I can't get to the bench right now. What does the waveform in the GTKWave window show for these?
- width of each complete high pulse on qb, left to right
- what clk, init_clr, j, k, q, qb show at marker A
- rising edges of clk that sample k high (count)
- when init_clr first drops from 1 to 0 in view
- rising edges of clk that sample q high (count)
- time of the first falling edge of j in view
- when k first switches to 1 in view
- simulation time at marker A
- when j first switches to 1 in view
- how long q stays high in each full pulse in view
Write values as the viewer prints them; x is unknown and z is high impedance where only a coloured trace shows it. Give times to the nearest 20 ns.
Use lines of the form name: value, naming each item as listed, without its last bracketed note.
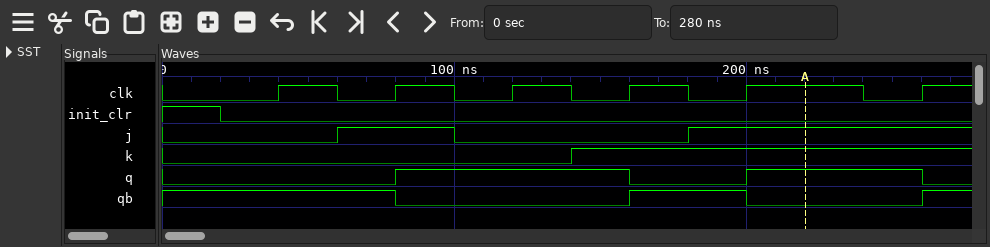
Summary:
width of each complete high pulse on qb, left to right: 40 ns
what clk, init_clr, j, k, q, qb show at marker A: clk=1, init_clr=0, j=1, k=1, q=1, qb=0
rising edges of clk that sample k high: 3
when init_clr first drops from 1 to 0 in view: 20 ns
rising edges of clk that sample q high: 3
time of the first falling edge of j in view: 100 ns
when k first switches to 1 in view: 140 ns
simulation time at marker A: 220 ns
when j first switches to 1 in view: 60 ns
how long q stays high in each full pulse in view: 80 ns, 60 ns
